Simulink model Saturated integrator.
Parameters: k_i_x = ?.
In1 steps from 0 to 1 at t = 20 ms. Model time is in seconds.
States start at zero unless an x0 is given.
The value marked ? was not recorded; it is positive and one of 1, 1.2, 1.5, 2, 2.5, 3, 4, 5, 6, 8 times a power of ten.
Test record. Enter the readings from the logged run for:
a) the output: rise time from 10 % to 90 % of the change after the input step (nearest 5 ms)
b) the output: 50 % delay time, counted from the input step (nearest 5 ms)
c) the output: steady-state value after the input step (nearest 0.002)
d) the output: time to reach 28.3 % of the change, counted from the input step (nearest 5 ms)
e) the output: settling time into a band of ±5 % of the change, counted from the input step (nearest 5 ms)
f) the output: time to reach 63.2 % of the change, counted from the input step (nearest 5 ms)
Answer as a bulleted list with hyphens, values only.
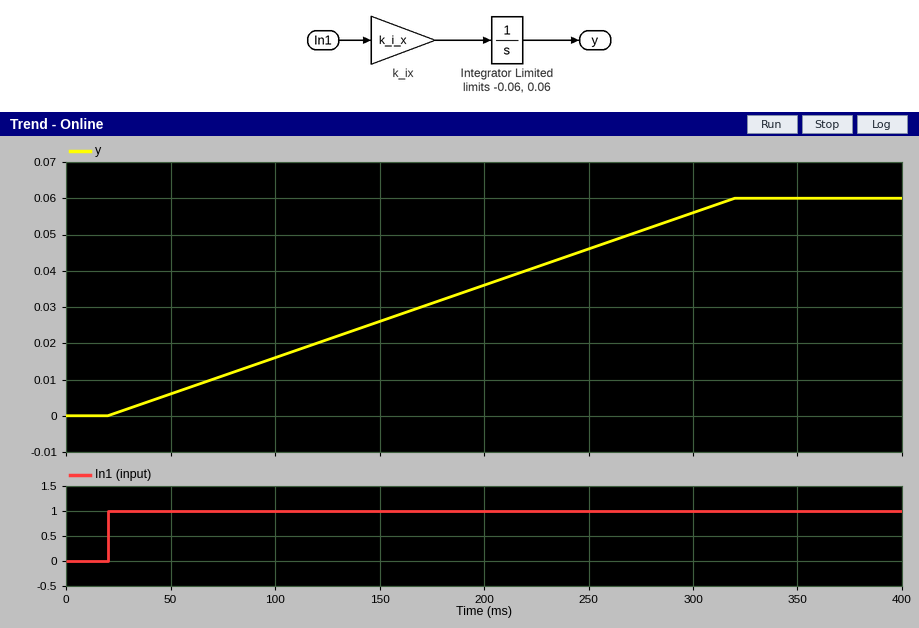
- 240 ms
- 150 ms
- 0.060
- 85 ms
- 285 ms
- 190 ms
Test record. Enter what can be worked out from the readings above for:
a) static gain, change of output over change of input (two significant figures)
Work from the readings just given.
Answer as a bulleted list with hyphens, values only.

- 0.060
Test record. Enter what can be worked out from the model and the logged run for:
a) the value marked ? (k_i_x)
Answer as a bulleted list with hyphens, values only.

- 0.2
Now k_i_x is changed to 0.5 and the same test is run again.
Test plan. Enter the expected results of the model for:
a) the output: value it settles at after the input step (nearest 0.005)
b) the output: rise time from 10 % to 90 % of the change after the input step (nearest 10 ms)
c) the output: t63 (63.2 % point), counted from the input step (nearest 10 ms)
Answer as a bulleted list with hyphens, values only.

- 0.060
- 100 ms
- 80 ms
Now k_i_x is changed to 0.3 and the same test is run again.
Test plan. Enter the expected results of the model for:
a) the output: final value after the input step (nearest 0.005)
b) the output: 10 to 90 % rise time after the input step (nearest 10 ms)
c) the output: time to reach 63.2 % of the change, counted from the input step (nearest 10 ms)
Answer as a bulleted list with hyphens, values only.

- 0.060
- 160 ms
- 130 ms
